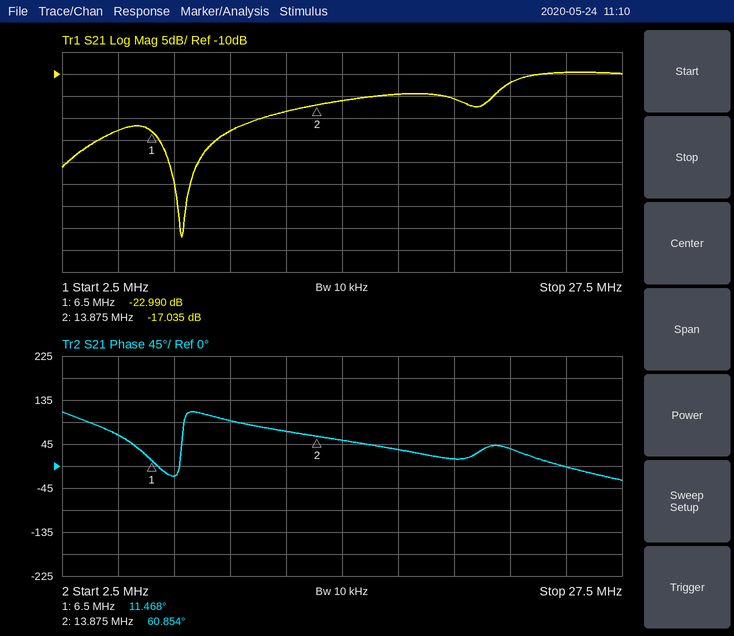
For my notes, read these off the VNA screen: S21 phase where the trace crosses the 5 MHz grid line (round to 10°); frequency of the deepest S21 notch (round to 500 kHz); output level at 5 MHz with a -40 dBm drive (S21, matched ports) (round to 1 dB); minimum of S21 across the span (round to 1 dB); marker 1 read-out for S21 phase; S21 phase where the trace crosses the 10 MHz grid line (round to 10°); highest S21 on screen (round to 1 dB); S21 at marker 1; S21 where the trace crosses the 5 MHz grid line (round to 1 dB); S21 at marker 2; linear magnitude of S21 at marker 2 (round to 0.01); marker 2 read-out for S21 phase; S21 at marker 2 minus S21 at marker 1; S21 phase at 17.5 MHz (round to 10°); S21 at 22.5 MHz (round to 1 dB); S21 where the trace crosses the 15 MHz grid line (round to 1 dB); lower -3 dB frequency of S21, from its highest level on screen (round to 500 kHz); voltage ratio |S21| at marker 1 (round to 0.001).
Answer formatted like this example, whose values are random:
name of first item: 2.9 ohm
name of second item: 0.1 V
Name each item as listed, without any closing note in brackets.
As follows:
S21 phase where the trace crosses the 5 MHz grid line: 60°
frequency of the deepest S21 notch: 8.0 MHz
output level at 5 MHz with a -40 dBm drive (S21, matched ports): -63 dBm
minimum of S21 across the span: -47 dB
marker 1 read-out for S21 phase: 11.468°
S21 phase where the trace crosses the 10 MHz grid line: 90°
highest S21 on screen: -10 dB
S21 at marker 1: -22.990 dB
S21 where the trace crosses the 5 MHz grid line: -23 dB
S21 at marker 2: -17.035 dB
linear magnitude of S21 at marker 2: 0.14
marker 2 read-out for S21 phase: 60.854°
S21 at marker 2 minus S21 at marker 1: 5.955 dB
S21 phase at 17.5 MHz: 30°
S21 at 22.5 MHz: -12 dB
S21 where the trace crosses the 15 MHz grid line: -16 dB
lower -3 dB frequency of S21, from its highest level on screen: 22.5 MHz
voltage ratio |S21| at marker 1: 0.071
